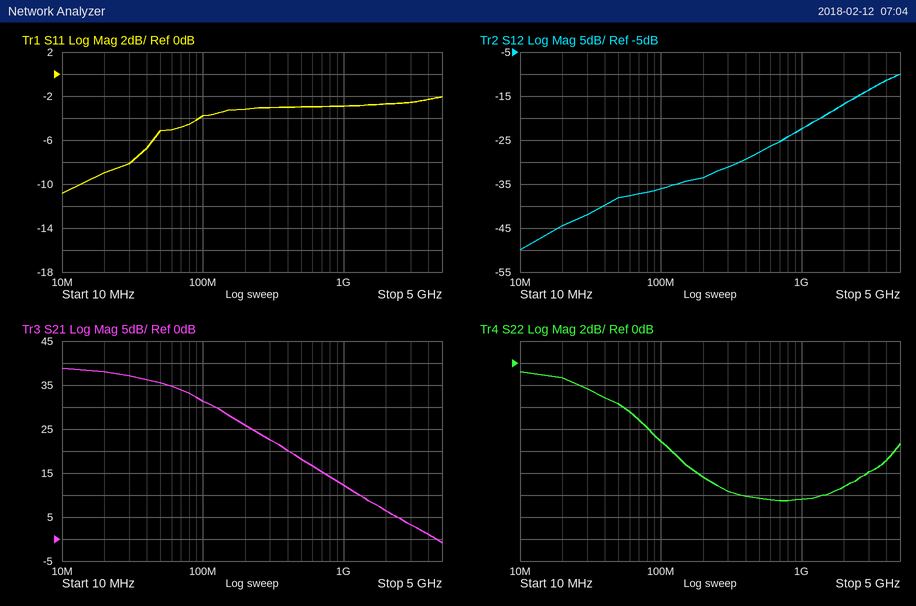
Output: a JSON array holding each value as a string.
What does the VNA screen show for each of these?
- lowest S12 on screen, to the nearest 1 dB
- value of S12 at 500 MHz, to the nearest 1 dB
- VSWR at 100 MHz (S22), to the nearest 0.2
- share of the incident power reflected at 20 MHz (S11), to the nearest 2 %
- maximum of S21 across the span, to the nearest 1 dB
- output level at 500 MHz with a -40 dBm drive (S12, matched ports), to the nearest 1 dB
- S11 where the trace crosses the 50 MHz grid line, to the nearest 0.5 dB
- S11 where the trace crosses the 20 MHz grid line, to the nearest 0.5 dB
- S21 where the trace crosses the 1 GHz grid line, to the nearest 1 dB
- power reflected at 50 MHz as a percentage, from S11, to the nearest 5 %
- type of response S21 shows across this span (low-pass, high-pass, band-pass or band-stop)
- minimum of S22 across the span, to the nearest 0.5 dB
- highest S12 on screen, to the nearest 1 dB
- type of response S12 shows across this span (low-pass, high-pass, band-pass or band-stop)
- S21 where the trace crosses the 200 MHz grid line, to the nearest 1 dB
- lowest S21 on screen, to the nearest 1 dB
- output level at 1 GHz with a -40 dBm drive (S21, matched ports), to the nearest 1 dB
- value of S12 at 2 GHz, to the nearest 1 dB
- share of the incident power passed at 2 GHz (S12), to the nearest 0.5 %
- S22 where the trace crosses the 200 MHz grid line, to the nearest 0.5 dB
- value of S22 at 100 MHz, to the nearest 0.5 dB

["-50 dB", "-28 dB", "2.6", "12 %", "39 dB", "-68 dBm", "-5.0 dB", "-9.0 dB", "12 dB", "30 %", "low-pass", "-12.5 dB", "-10 dB", "high-pass", "26 dB", "-1 dB", "-28 dBm", "-17 dB", "2.0 %", "-10.5 dB", "-7.0 dB"]
